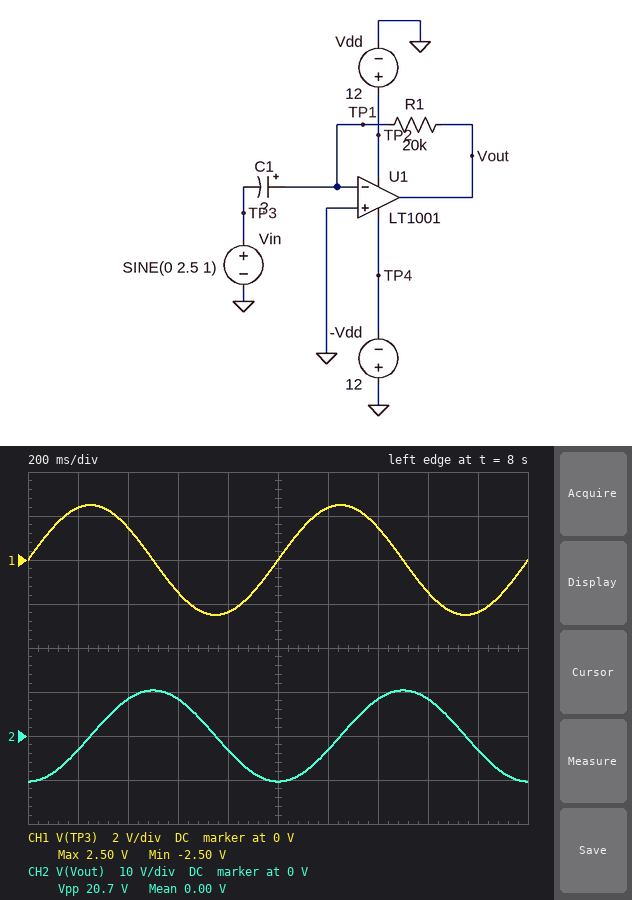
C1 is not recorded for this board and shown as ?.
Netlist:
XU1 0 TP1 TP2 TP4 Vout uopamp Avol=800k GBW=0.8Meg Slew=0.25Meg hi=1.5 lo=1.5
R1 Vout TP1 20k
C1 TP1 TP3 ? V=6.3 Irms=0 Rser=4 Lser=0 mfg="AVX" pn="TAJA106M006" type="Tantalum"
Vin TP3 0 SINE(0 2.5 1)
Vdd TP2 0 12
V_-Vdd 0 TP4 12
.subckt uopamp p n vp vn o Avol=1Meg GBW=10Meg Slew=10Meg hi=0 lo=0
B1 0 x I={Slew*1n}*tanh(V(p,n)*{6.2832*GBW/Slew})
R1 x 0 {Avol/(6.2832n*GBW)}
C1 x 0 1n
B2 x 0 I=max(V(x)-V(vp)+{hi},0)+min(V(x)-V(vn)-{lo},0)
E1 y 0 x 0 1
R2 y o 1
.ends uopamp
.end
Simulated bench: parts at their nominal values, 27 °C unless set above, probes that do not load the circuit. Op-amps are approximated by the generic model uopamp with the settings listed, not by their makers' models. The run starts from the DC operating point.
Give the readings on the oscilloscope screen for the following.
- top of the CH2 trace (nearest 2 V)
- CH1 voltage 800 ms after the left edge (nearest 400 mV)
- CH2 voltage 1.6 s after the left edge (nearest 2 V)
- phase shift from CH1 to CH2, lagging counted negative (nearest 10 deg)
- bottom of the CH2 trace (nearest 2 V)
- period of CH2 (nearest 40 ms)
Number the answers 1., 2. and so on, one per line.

1. 10 V
2. -2.4 V
3. 8 V
4. -90 deg
5. -10 V
6. 1.00 s
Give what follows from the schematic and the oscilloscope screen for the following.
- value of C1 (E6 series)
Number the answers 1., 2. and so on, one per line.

1. 33 µF
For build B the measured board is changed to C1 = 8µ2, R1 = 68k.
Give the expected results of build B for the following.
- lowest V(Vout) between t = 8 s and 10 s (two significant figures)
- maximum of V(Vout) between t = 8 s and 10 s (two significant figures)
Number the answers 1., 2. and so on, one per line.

1. -8.8 V
2. 8.8 V
